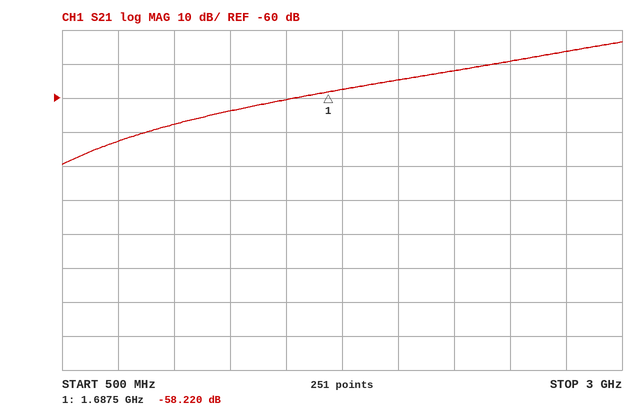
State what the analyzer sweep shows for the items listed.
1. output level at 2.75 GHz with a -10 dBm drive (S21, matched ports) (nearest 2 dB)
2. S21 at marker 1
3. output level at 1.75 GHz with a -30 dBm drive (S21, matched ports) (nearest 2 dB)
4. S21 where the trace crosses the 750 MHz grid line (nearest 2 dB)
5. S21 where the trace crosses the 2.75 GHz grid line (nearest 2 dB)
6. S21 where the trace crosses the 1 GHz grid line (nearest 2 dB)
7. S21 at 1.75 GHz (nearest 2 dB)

-56 dBm
-58.220 dB
-88 dBm
-72 dB
-46 dB
-68 dB
-58 dB
